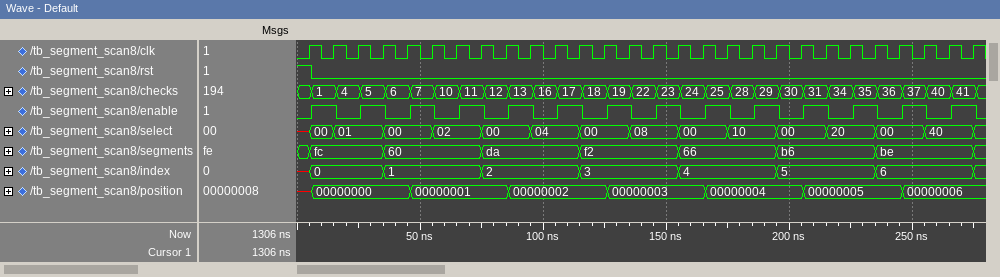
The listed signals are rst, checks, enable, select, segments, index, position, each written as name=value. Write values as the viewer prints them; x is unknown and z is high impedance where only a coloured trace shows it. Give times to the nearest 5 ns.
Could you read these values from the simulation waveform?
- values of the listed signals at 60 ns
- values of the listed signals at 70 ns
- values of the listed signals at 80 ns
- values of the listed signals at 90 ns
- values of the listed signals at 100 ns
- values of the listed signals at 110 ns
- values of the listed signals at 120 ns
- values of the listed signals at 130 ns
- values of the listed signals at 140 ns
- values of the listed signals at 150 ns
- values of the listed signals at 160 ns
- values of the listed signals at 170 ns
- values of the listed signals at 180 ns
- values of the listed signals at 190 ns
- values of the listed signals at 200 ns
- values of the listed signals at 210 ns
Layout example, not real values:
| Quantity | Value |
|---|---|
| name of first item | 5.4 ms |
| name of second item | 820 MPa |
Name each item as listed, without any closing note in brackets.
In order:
| Quantity | Value |
|---|---|
| values of the listed signals at 60 ns | rst=0, checks=10, enable=0, select=02, segments=60, index=1, position=00000001 |
| values of the listed signals at 70 ns | rst=0, checks=11, enable=1, select=02, segments=60, index=1, position=00000001 |
| values of the listed signals at 80 ns | rst=0, checks=12, enable=0, select=00, segments=da, index=2, position=00000001 |
| values of the listed signals at 90 ns | rst=0, checks=13, enable=1, select=00, segments=da, index=2, position=00000002 |
| values of the listed signals at 100 ns | rst=0, checks=16, enable=0, select=04, segments=da, index=2, position=00000002 |
| values of the listed signals at 110 ns | rst=0, checks=17, enable=1, select=04, segments=da, index=2, position=00000002 |
| values of the listed signals at 120 ns | rst=0, checks=18, enable=0, select=00, segments=f2, index=3, position=00000002 |
| values of the listed signals at 130 ns | rst=0, checks=19, enable=1, select=00, segments=f2, index=3, position=00000003 |
| values of the listed signals at 140 ns | rst=0, checks=22, enable=0, select=08, segments=f2, index=3, position=00000003 |
| values of the listed signals at 150 ns | rst=0, checks=23, enable=1, select=08, segments=f2, index=3, position=00000003 |
| values of the listed signals at 160 ns | rst=0, checks=24, enable=0, select=00, segments=66, index=4, position=00000003 |
| values of the listed signals at 170 ns | rst=0, checks=25, enable=1, select=00, segments=66, index=4, position=00000004 |
| values of the listed signals at 180 ns | rst=0, checks=28, enable=0, select=10, segments=66, index=4, position=00000004 |
| values of the listed signals at 190 ns | rst=0, checks=29, enable=1, select=10, segments=66, index=4, position=00000004 |
| values of the listed signals at 200 ns | rst=0, checks=30, enable=0, select=00, segments=b6, index=5, position=00000004 |
| values of the listed signals at 210 ns | rst=0, checks=31, enable=1, select=00, segments=b6, index=5, position=00000005 |
